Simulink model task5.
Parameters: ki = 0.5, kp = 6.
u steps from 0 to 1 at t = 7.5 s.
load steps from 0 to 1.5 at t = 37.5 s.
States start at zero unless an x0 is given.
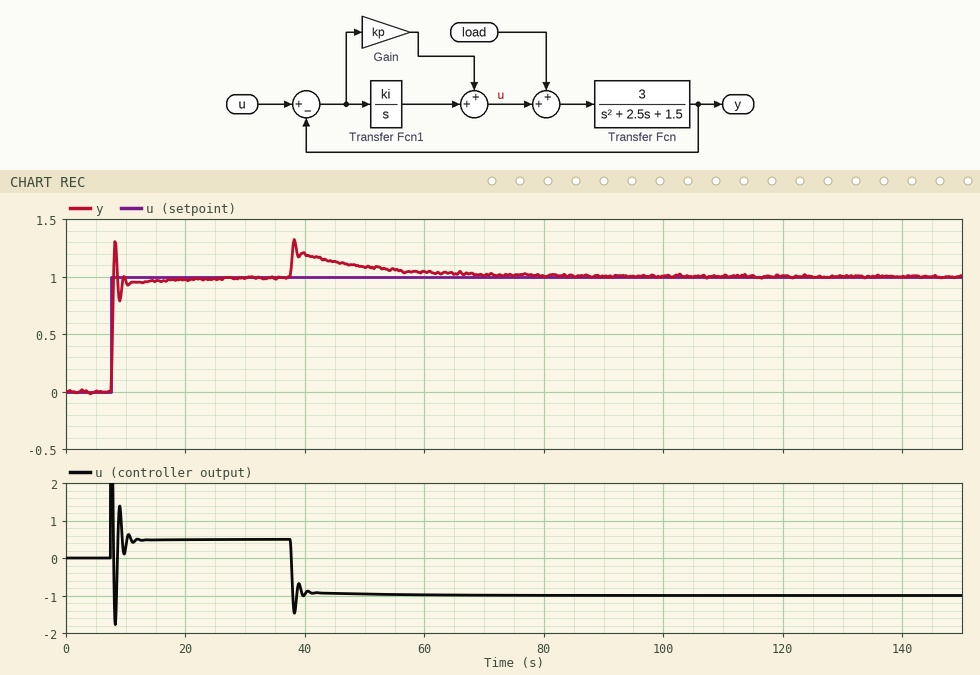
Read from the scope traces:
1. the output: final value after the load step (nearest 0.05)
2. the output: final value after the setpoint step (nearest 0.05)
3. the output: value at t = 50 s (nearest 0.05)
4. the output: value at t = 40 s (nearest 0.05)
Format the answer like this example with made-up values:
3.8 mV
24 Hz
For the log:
1.00
1.00
1.10
1.20
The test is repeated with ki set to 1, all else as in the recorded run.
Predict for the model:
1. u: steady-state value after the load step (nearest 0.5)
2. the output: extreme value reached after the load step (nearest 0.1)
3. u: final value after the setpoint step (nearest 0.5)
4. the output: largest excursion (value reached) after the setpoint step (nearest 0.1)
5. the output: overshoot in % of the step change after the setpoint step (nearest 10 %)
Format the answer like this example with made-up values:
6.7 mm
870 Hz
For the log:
-1.0
1.3
0.5
1.3
30 %
